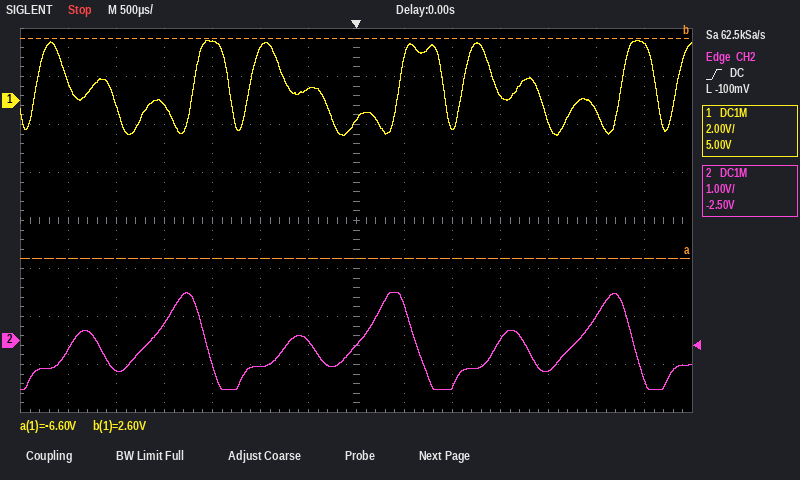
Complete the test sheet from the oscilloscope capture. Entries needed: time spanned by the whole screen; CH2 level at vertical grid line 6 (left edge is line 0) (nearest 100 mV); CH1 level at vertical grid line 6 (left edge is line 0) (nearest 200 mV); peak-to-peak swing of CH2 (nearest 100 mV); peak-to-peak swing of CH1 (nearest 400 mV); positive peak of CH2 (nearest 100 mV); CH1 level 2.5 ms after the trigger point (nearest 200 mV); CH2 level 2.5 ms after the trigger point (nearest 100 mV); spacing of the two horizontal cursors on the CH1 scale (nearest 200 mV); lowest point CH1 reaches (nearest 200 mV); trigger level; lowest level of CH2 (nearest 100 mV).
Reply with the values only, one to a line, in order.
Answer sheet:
7 ms
0.0 V
400 mV
2.0 V
4.0 V
1.0 V
-400 mV
500 mV
9.2 V
-1.4 V
-100 mV
-1.0 V
